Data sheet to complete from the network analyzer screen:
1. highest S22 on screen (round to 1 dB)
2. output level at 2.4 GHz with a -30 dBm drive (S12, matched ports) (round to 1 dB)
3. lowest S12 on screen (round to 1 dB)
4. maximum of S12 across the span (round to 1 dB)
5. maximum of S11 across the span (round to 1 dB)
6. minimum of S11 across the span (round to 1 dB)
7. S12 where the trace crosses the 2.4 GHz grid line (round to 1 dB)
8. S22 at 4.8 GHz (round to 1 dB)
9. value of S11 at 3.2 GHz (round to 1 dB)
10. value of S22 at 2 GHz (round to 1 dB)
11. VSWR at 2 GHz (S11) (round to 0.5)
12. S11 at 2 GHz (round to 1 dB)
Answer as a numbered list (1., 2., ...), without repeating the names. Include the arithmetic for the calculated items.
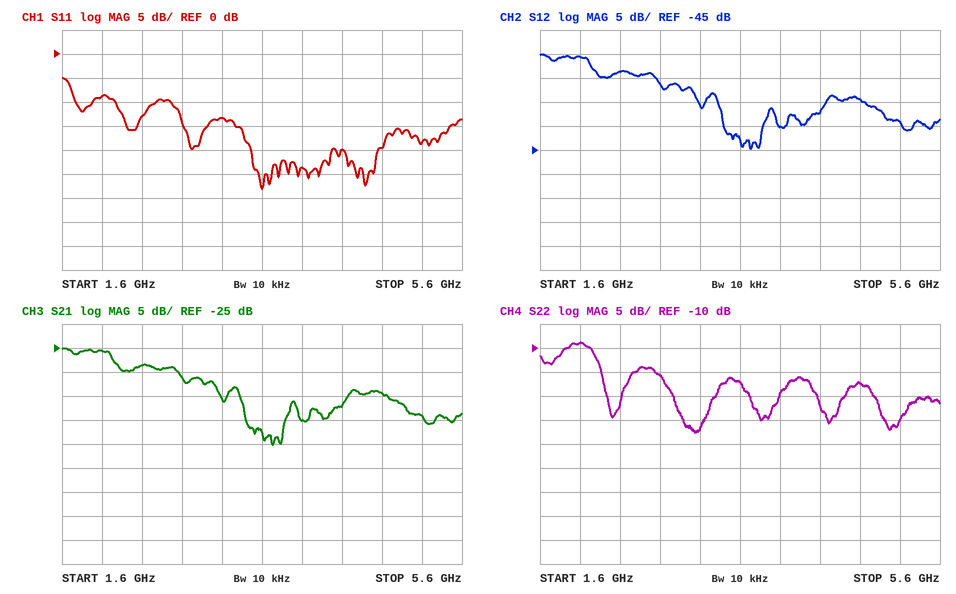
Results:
1. -9 dB
2. -30 dBm + (-29 dB) = -59 dBm
3. -45 dB
4. -25 dB
5. -5 dB
6. -28 dB
7. -29 dB
8. -17 dB
9. -13 dB
10. -9 dB
11. |Γ| = 10^(-9/20) = 0.3548; VSWR = (1 + 0.3548)/(1 − 0.3548) ≈ 2.10, so 2.0 to the nearest 0.5
12. -9 dB
